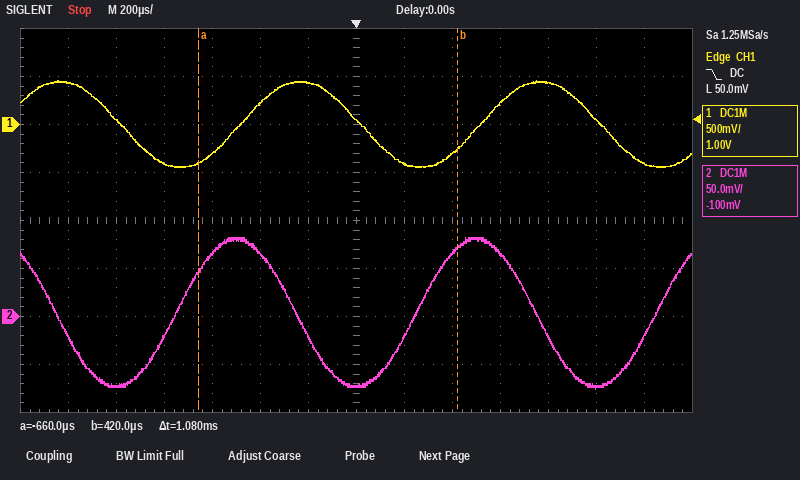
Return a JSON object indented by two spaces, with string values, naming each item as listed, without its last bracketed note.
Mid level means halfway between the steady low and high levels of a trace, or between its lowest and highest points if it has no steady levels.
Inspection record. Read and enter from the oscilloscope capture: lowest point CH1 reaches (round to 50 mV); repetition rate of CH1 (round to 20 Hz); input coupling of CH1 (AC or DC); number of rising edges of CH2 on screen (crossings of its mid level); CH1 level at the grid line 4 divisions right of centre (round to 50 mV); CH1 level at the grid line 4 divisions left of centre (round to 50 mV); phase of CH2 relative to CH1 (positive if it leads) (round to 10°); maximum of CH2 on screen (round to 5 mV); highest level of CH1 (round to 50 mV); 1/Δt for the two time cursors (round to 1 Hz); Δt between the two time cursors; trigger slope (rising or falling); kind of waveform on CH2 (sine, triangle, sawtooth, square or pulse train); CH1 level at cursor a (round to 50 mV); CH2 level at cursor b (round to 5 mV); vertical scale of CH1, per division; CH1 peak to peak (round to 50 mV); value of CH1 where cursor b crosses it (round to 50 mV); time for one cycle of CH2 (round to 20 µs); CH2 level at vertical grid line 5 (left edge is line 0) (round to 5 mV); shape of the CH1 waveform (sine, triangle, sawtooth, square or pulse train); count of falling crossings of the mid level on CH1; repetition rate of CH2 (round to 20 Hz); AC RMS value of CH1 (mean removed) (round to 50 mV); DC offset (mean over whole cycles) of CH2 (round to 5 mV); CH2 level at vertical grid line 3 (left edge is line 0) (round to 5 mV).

{
  "lowest point CH1 reaches": "-450 mV",
  "repetition rate of CH1": "1.00 kHz",
  "input coupling of CH1": "DC",
  "number of rising edges of CH2 on screen": "3",
  "CH1 level at the grid line 4 divisions right of centre": "450 mV",
  "CH1 level at the grid line 4 divisions left of centre": "-400 mV",
  "phase of CH2 relative to CH1 (positive if it leads)": "+100°",
  "maximum of CH2 on screen": "80 mV",
  "highest level of CH1": "450 mV",
  "1/Δt for the two time cursors": "926 Hz",
  "Δt between the two time cursors": "1.08 ms",
  "trigger slope": "falling",
  "kind of waveform on CH2": "sine",
  "CH1 level at cursor a": "-400 mV",
  "CH2 level at cursor b": "70 mV",
  "vertical scale of CH1, per division": "500 mV",
  "CH1 peak to peak": "900 mV",
  "value of CH1 where cursor b crosses it": "-250 mV",
  "time for one cycle of CH2": "1.00 ms",
  "CH2 level at vertical grid line 5 (left edge is line 0)": "65 mV",
  "shape of the CH1 waveform": "sine",
  "count of falling crossings of the mid level on CH1": "3",
  "repetition rate of CH2": "1.00 kHz",
  "AC RMS value of CH1 (mean removed)": "300 mV",
  "DC offset (mean over whole cycles) of CH2": "5 mV",
  "CH2 level at vertical grid line 3 (left edge is line 0)": "-20 mV"
}
